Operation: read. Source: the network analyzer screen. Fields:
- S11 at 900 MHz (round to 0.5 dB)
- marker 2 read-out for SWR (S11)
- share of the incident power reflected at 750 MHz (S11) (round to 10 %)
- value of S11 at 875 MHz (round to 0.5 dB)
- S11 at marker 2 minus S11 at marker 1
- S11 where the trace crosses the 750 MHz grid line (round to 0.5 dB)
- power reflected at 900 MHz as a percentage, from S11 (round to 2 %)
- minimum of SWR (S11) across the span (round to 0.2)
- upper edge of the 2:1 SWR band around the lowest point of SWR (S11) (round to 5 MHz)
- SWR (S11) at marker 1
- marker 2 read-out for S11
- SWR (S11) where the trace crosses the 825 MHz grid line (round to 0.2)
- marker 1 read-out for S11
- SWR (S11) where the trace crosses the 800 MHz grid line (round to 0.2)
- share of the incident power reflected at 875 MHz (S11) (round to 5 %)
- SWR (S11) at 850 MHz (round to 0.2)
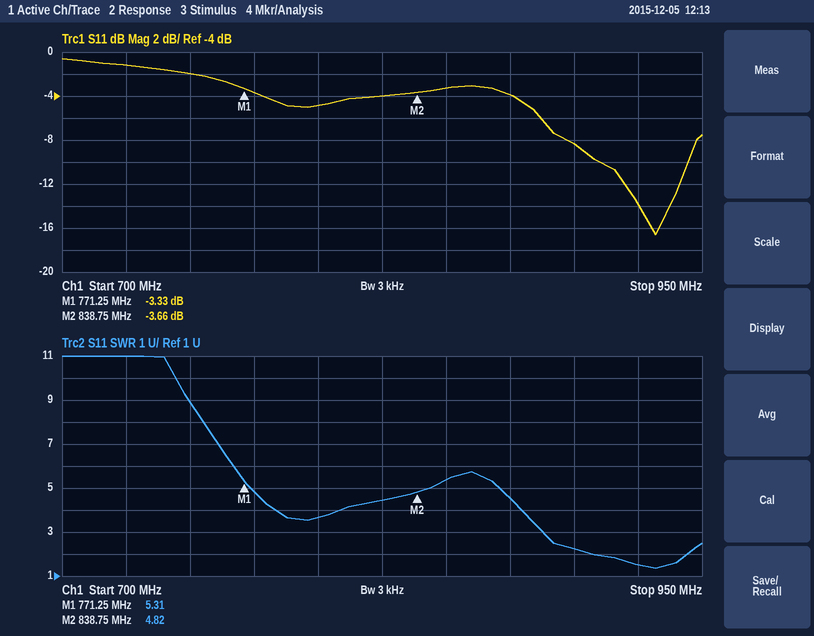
-8.5 dB
4.82
60 %
-4.0 dB
-0.33 dB
-2.0 dB
14 %
1.4
945 MHz
5.31
-3.66 dB
4.4
-3.33 dB
3.6
40 %
5.4
